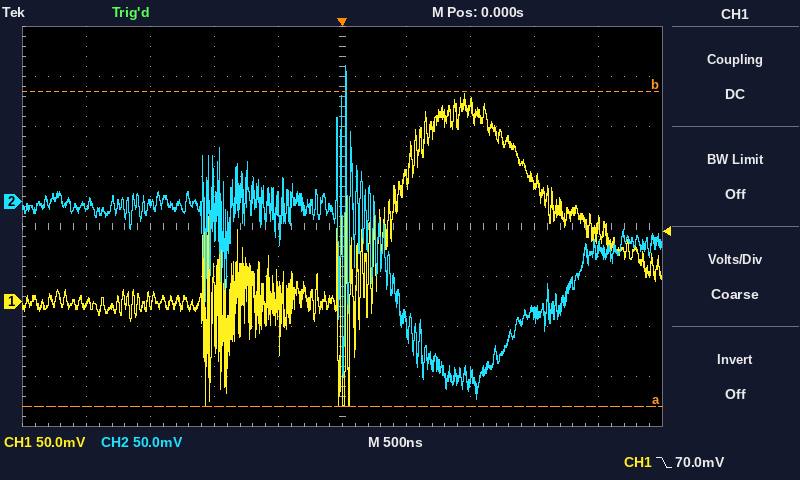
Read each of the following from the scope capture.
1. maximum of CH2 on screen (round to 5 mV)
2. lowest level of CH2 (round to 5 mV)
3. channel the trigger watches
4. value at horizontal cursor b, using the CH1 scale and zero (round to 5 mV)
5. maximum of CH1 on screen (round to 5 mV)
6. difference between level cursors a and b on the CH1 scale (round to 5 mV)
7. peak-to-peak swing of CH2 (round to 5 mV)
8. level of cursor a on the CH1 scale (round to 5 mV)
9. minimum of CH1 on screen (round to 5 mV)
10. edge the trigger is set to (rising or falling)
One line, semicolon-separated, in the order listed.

135 mV; -200 mV; CH1; 210 mV; 210 mV; 315 mV; 335 mV; -105 mV; -105 mV; falling
